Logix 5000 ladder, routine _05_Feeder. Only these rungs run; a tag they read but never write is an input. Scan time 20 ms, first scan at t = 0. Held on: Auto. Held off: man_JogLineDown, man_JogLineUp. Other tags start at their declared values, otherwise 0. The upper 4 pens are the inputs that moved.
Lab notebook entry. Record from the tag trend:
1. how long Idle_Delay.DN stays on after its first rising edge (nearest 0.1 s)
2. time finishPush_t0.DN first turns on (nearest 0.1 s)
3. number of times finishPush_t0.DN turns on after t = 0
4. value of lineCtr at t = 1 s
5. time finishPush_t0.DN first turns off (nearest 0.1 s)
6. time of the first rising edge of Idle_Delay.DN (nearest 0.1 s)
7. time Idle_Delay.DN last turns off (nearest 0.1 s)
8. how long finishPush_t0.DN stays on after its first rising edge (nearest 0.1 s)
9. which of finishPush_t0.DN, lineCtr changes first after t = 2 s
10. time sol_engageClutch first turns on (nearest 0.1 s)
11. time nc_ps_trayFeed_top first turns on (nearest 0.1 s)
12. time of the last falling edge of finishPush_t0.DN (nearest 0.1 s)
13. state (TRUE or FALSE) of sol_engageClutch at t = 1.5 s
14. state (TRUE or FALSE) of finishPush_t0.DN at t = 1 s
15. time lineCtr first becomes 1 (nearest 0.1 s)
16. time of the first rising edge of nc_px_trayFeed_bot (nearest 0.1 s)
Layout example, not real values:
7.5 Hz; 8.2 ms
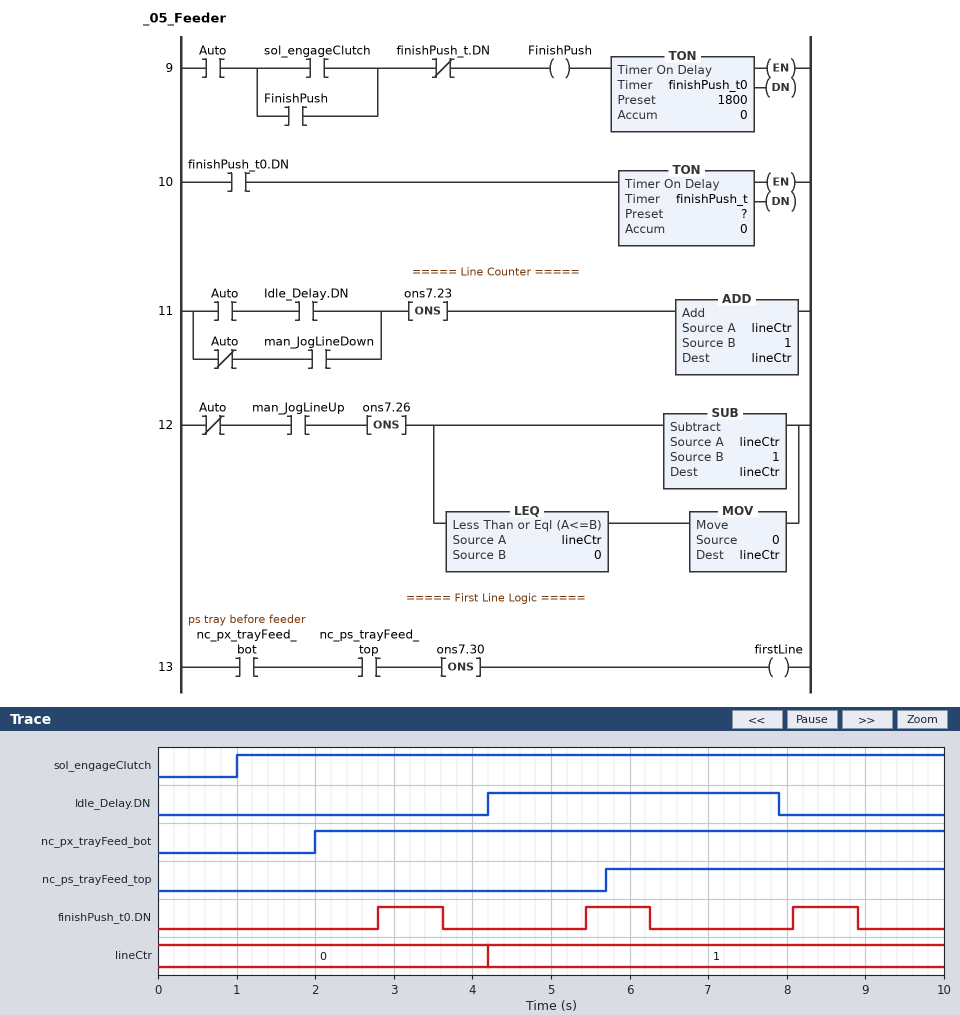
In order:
3.7 s; 2.8 s; 3; 0; 3.6 s; 4.2 s; 7.9 s; 0.8 s; finishPush_t0.DN; 1.0 s; 5.7 s; 8.9 s; TRUE; FALSE; 4.2 s; 2.0 s
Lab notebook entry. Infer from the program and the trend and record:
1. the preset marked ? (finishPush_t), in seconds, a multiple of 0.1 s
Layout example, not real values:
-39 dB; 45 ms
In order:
0.8 s
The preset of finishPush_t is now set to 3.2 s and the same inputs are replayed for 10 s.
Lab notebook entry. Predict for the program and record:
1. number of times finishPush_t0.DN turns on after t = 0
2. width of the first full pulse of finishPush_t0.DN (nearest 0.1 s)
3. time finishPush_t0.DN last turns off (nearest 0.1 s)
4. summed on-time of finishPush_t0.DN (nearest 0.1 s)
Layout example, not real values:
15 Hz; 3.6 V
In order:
2; 3.2 s; 6.0 s; 5.4 s
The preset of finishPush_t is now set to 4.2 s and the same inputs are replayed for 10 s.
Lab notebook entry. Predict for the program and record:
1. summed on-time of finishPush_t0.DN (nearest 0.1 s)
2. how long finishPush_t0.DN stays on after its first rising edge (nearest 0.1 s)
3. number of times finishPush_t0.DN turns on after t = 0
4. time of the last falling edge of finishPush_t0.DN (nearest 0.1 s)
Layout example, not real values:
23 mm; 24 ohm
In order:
5.4 s; 4.2 s; 2; 7.0 s
